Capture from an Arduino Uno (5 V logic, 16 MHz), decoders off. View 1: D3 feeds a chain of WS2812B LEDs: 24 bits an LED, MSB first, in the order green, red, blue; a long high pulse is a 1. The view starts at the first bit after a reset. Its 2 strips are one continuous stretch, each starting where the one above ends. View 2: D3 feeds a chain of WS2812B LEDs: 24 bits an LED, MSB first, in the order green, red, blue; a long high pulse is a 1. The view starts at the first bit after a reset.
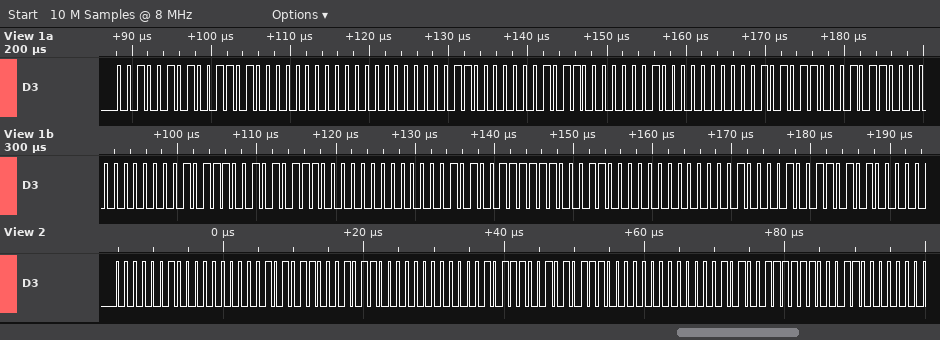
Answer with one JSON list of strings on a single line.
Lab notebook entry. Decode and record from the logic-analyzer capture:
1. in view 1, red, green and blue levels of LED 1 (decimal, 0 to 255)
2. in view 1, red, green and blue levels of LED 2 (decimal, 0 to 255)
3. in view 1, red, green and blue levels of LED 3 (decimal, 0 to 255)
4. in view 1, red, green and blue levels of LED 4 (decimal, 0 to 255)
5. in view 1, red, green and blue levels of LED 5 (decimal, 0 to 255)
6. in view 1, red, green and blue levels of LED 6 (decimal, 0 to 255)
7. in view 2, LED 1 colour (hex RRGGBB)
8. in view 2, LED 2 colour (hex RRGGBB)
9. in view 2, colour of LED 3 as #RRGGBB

["52, 37, 0", "48, 0, 22", "0, 2, 86", "0, 44, 46", "0, 87, 5", "24, 63, 0", "#000256", "#002C2E", "#005705"]
